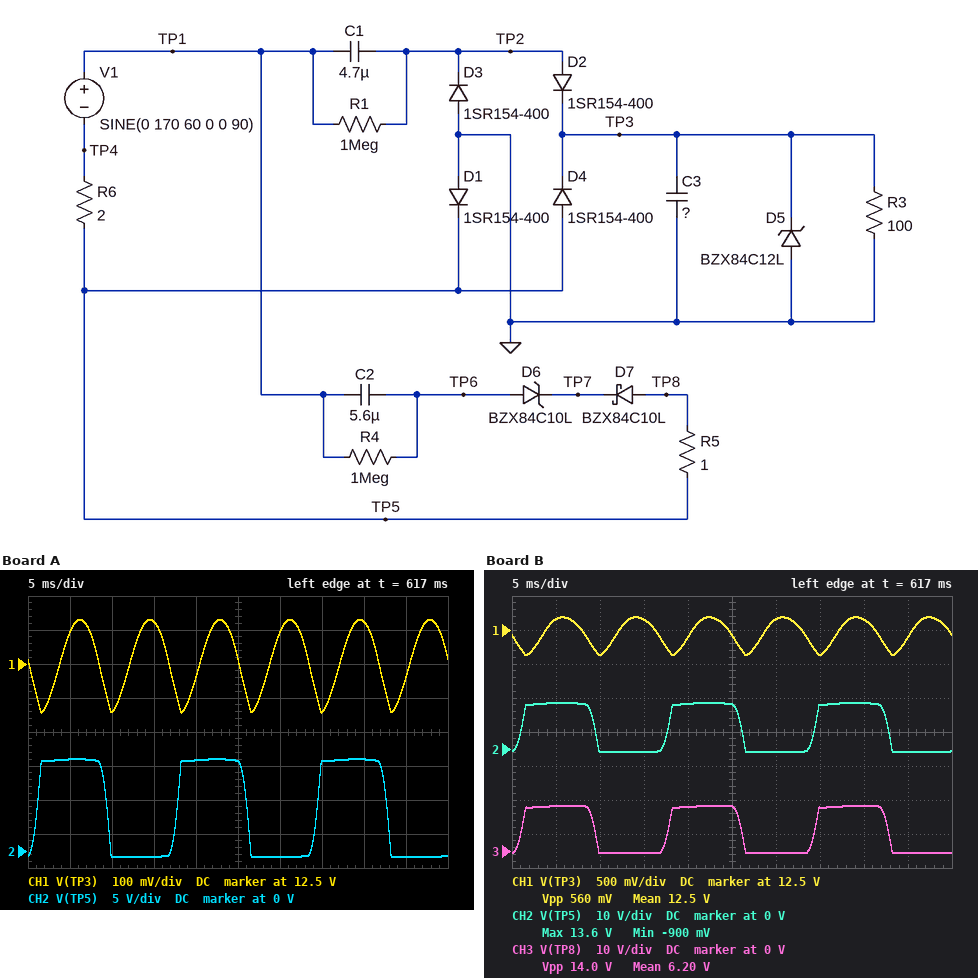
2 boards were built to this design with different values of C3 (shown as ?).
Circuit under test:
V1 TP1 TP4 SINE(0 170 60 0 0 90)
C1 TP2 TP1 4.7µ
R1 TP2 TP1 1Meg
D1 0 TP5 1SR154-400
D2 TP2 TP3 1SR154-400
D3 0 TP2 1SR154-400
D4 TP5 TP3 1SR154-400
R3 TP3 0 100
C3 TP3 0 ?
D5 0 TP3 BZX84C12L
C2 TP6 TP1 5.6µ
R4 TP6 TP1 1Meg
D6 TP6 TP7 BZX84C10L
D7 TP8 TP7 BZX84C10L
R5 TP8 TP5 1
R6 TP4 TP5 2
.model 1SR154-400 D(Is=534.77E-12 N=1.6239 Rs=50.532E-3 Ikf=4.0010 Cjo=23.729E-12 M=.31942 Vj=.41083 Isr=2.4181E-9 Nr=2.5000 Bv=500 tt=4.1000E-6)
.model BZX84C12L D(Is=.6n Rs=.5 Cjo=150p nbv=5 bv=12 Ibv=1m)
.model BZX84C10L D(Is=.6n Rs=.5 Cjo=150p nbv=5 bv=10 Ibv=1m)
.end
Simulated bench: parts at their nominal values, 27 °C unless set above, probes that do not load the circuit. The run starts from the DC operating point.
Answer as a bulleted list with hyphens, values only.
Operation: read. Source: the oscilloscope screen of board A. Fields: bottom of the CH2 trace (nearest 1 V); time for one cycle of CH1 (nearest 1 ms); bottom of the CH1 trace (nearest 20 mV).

- -1 V
- 8 ms
- 12.36 V
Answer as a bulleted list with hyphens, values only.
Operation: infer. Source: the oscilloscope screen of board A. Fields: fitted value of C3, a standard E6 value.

- 1.5 mF
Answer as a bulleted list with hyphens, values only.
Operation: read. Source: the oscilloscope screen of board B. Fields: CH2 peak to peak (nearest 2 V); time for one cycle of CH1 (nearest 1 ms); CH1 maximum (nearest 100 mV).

- 14 V
- 8 ms
- 12.7 V
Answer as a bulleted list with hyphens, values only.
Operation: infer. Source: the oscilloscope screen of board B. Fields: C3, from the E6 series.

- 680 µF
